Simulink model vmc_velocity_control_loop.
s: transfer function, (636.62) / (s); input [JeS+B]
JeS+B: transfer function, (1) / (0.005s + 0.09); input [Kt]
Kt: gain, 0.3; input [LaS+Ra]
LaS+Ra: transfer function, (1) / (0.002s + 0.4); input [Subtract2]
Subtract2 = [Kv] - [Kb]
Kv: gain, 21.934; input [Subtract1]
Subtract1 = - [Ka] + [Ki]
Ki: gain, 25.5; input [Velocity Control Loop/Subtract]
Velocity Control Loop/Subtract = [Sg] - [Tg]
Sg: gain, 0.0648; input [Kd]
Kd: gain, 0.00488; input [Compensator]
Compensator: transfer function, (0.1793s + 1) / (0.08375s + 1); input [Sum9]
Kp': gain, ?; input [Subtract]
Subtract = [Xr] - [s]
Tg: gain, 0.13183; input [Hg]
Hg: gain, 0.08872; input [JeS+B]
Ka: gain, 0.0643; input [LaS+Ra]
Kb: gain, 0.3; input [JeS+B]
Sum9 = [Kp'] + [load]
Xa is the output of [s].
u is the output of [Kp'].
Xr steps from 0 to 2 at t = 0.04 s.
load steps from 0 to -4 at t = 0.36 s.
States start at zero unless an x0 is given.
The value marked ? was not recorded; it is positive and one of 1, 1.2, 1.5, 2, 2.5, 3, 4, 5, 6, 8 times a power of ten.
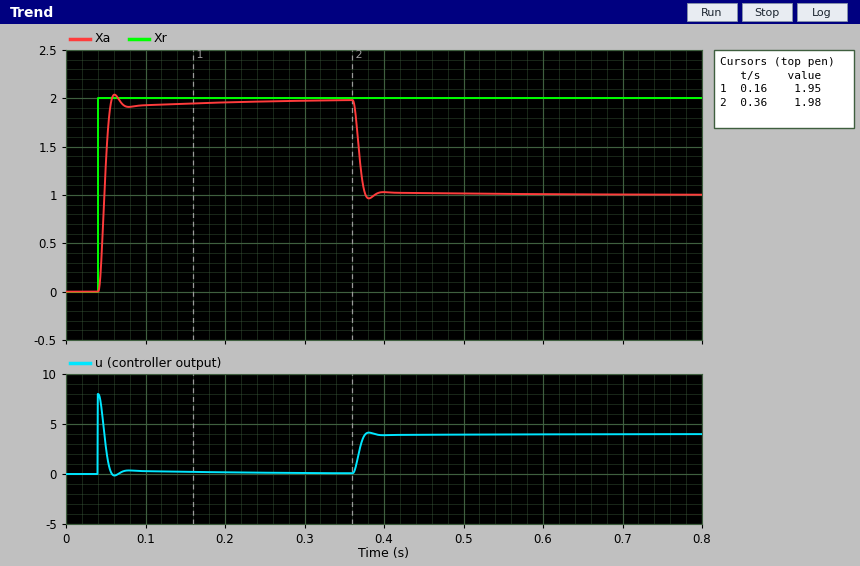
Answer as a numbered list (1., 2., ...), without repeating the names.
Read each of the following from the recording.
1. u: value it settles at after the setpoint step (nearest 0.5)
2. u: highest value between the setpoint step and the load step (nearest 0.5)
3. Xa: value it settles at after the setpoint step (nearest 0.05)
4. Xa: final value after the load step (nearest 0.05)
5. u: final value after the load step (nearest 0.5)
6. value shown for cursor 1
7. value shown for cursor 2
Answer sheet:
1. 0.0
2. 8.0
3. 2.00
4. 1.00
5. 4.0
6. 1.95
7. 1.98
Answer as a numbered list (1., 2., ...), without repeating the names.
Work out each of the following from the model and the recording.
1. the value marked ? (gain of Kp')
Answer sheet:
1. 4
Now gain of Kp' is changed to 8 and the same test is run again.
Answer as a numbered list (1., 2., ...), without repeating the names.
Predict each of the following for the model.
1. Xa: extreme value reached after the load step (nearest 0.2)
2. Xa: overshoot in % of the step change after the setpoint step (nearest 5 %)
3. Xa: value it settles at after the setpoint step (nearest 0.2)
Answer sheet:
1. 1.4
2. 25 %
3. 2.0
